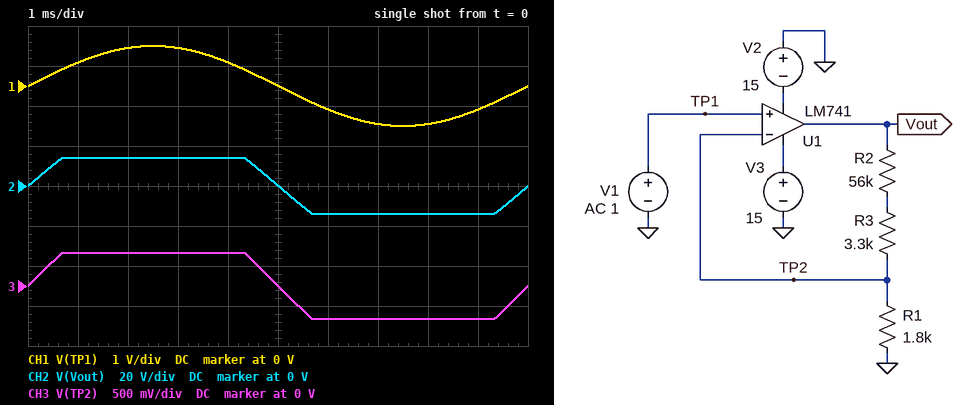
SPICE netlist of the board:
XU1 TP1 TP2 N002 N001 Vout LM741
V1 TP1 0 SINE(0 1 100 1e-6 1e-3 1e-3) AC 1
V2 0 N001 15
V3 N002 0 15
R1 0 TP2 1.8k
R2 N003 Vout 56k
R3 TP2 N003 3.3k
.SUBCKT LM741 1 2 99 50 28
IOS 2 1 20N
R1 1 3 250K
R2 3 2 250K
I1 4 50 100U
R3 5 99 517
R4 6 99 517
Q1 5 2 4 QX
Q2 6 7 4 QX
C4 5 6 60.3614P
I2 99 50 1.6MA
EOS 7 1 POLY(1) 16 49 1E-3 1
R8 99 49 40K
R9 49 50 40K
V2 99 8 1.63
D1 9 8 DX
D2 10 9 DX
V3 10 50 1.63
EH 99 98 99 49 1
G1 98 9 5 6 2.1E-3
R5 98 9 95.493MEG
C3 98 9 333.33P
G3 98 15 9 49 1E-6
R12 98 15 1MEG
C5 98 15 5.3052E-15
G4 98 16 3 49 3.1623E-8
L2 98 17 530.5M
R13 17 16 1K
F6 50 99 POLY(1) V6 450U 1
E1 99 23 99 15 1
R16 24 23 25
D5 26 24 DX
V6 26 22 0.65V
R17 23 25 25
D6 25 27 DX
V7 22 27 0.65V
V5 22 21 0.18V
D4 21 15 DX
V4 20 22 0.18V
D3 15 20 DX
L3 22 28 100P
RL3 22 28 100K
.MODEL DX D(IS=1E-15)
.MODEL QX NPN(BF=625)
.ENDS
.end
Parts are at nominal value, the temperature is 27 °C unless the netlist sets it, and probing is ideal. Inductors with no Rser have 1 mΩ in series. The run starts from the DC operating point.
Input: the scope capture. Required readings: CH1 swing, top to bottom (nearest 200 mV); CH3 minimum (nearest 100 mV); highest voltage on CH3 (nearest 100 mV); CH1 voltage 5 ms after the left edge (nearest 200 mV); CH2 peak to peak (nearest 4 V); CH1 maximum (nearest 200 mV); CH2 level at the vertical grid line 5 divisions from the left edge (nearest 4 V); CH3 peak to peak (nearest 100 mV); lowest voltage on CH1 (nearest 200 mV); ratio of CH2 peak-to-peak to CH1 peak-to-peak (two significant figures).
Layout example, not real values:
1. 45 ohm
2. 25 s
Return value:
1. 2.0 V
2. -400 mV
3. 400 mV
4. 0 V
5. 28 V
6. 1.0 V
7. 0 V
8. 800 mV
9. -1.0 V
10. 14
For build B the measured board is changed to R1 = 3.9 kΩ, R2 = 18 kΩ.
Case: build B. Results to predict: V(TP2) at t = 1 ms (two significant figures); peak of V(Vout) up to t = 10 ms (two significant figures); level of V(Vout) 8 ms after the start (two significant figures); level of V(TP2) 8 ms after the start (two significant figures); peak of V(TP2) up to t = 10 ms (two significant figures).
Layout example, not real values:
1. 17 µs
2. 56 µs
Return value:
1. 590 mV
2. 6.5 V
3. -6.1 V
4. -950 mV
5. 1.0 V
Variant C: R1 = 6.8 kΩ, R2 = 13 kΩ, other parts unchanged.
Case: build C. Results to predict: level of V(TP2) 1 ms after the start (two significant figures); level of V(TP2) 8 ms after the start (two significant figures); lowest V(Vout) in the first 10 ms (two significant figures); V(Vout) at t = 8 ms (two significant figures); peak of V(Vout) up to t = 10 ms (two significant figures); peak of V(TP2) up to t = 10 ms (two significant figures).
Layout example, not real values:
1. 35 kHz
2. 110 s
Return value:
1. 590 mV
2. -950 mV
3. -3.4 V
4. -3.2 V
5. 3.4 V
6. 1.0 V
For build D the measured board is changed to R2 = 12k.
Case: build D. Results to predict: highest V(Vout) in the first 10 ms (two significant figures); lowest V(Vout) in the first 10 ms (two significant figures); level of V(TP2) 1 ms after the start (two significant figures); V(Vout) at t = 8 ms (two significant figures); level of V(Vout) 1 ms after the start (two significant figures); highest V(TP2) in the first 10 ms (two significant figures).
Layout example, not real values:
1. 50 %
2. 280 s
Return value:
1. 9.5 V
2. -9.5 V
3. 590 mV
4. -9.0 V
5. 5.6 V
6. 1.0 V
